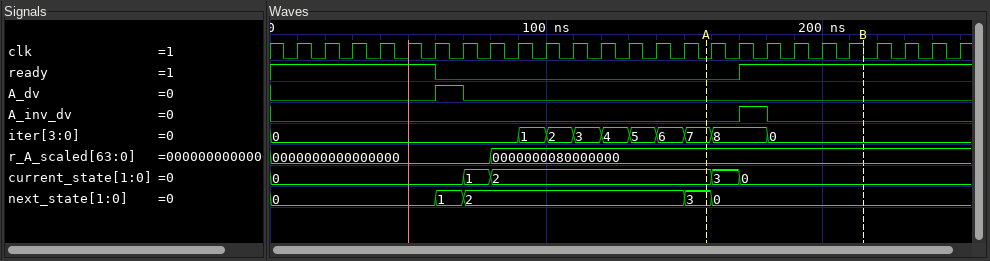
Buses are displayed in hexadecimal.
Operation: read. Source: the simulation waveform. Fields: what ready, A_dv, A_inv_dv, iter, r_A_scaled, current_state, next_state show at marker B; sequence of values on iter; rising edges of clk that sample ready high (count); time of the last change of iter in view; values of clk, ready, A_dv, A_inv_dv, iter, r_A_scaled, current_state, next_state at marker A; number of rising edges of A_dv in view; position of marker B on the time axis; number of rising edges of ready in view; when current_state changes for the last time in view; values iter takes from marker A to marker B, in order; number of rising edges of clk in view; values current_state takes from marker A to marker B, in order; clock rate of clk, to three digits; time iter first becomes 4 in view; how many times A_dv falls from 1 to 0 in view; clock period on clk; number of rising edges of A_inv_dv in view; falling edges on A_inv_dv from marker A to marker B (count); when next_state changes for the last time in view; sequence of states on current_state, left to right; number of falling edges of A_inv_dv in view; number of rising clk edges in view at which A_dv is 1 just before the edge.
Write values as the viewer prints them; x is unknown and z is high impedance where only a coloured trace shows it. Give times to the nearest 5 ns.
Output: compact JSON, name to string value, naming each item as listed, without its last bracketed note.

{"what ready, A_dv, A_inv_dv, iter, r_A_scaled, current_state, next_state show at marker B": "ready=1, A_dv=0, A_inv_dv=0, iter=0, r_A_scaled=0000000080000000, current_state=0, next_state=0", "sequence of values on iter": "0, 1, 2, 3, 4, 5, 6, 7, 8, 0", "rising edges of clk that sample ready high": "14", "time of the last change of iter in view": "180 ns", "values of clk, ready, A_dv, A_inv_dv, iter, r_A_scaled, current_state, next_state at marker A": "clk=0, ready=0, A_dv=0, A_inv_dv=0, iter=7, r_A_scaled=0000000080000000, current_state=2, next_state=3", "number of rising edges of A_dv in view": "1", "position of marker B on the time axis": "215 ns", "number of rising edges of ready in view": "1", "when current_state changes for the last time in view": "170 ns", "values iter takes from marker A to marker B, in order": "7, 8, 0", "number of rising edges of clk in view": "25", "values current_state takes from marker A to marker B, in order": "2, 3, 0", "clock rate of clk, to three digits": "100 MHz", "time iter first becomes 4 in view": "120 ns", "how many times A_dv falls from 1 to 0 in view": "1", "clock period on clk": "10 ns", "number of rising edges of A_inv_dv in view": "1", "falling edges on A_inv_dv from marker A to marker B": "1", "when next_state changes for the last time in view": "160 ns", "sequence of states on current_state, left to right": "0, 1, 2, 3, 0", "number of falling edges of A_inv_dv in view": "1", "number of rising clk edges in view at which A_dv is 1 just before the edge": "1"}
